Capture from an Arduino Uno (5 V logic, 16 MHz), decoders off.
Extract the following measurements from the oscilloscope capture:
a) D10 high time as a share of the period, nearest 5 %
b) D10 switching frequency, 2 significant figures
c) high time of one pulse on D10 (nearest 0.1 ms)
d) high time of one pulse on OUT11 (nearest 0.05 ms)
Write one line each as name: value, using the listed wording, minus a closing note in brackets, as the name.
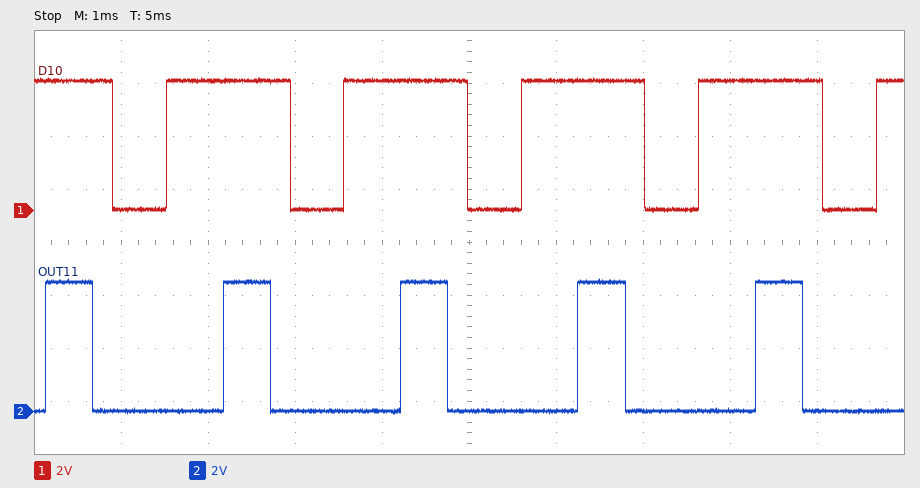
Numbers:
D10 high time as a share of the period, nearest 5 %: 70 %
D10 switching frequency, 2 significant figures: 490 Hz
high time of one pulse on D10: 1.4 ms
high time of one pulse on OUT11: 0.55 ms
